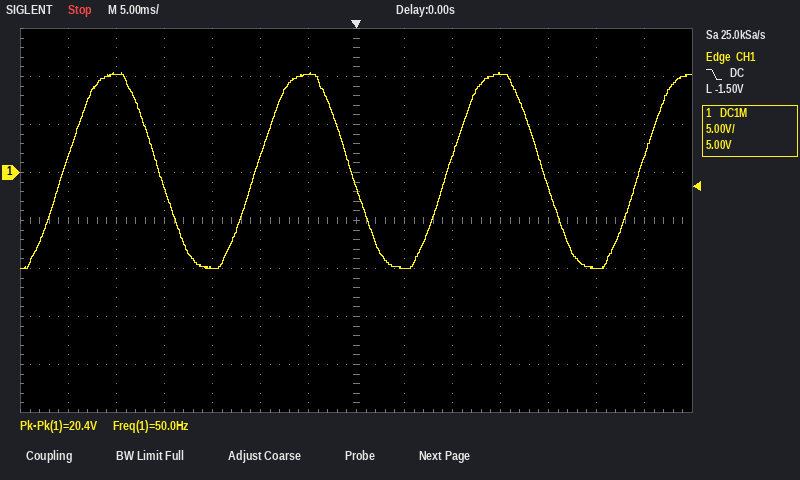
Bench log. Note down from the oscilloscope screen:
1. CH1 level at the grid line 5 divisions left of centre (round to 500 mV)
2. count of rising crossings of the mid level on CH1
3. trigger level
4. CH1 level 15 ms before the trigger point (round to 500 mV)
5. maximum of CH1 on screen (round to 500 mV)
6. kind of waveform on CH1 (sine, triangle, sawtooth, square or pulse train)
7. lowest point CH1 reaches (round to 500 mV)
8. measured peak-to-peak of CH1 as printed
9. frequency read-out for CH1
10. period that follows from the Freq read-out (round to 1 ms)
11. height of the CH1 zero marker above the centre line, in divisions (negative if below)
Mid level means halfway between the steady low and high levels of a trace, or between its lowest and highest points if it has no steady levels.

10.0 V
4
-1.50 V
-10.0 V
10.5 V
sine
-10.0 V
20.4 V
50.0 Hz
20 ms
+1.0 div
